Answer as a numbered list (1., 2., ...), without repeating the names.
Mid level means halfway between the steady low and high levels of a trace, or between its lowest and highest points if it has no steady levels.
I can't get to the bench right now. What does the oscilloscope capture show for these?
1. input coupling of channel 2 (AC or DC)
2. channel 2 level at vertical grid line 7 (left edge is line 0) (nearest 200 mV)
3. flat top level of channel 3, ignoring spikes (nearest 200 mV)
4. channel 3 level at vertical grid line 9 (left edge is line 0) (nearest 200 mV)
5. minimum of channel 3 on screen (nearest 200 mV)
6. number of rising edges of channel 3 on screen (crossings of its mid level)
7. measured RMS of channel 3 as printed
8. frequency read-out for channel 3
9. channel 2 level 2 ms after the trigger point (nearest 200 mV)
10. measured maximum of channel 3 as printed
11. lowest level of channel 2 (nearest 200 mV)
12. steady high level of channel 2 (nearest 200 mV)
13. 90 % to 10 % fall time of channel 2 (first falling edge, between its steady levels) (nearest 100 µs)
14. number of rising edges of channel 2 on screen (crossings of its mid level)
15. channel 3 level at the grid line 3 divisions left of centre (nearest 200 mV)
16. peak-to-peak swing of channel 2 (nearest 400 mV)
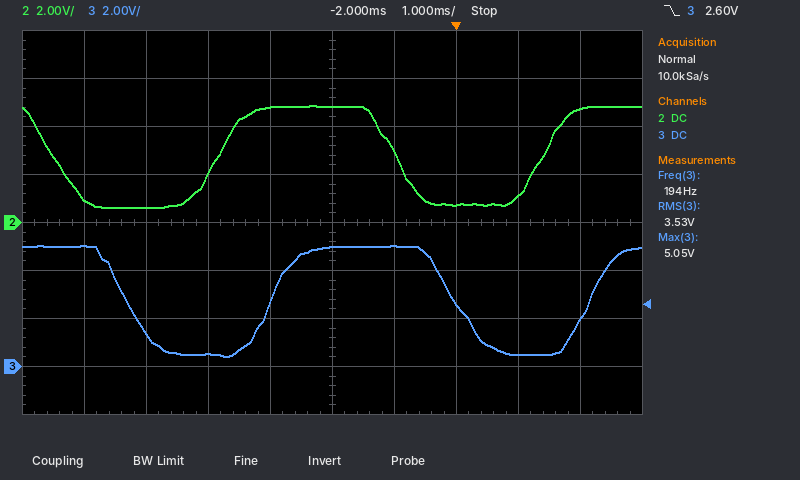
1. DC
2. 800 mV
3. 5.0 V
4. 2.0 V
5. 400 mV
6. 2
7. 3.53 V
8. 194 Hz
9. 4.8 V
10. 5.05 V
11. 600 mV
12. 4.8 V
13. 800 µs
14. 2
15. 1.4 V
16. 4.4 V
